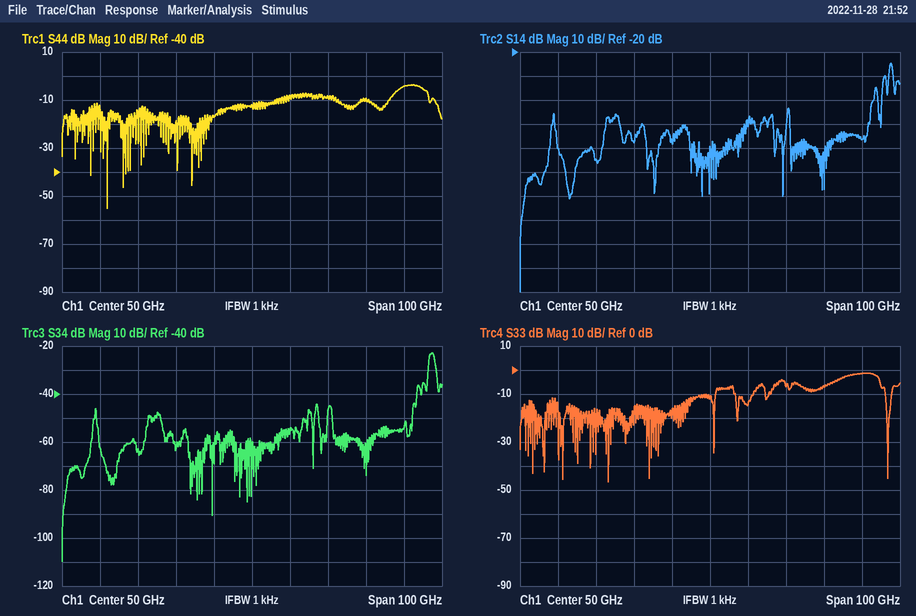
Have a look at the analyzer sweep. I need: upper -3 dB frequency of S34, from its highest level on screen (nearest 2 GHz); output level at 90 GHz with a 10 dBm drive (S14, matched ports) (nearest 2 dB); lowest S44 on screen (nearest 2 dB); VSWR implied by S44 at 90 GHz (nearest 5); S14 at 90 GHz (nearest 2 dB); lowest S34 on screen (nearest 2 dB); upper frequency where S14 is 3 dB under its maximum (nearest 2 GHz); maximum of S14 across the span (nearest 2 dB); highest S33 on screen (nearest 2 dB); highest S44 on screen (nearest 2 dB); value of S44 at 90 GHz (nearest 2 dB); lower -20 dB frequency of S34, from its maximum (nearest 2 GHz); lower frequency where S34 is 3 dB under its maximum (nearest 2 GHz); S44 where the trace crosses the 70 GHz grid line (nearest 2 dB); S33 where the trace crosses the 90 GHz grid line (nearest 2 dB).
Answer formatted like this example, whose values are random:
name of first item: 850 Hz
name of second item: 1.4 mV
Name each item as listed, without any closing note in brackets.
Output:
upper -3 dB frequency of S34, from its highest level on screen: 98 GHz
output level at 90 GHz with a 10 dBm drive (S14, matched ports): -46 dBm
lowest S44 on screen: -56 dB
VSWR implied by S44 at 90 GHz: 5
S14 at 90 GHz: -56 dB
lowest S34 on screen: -110 dB
upper frequency where S14 is 3 dB under its maximum: 98 GHz
maximum of S14 across the span: -24 dB
highest S33 on screen: -2 dB
highest S44 on screen: -4 dB
value of S44 at 90 GHz: -4 dB
lower -20 dB frequency of S34, from its maximum: 94 GHz
lower frequency where S34 is 3 dB under its maximum: 96 GHz
S44 where the trace crosses the 70 GHz grid line: -8 dB
S33 where the trace crosses the 90 GHz grid line: -2 dB
